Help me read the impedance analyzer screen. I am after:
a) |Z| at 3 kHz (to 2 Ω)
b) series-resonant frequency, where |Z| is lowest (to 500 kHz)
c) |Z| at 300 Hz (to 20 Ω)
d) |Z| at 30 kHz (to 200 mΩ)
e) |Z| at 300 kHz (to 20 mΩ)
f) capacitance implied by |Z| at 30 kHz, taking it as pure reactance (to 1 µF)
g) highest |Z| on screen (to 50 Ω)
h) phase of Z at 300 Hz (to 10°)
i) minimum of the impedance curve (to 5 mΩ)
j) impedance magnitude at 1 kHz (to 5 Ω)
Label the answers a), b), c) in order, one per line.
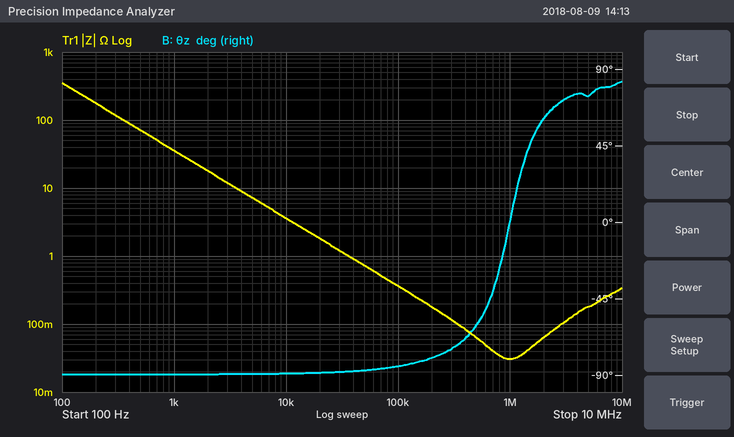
a) 12 Ω
b) 1.0 MHz
c) 120 Ω
d) 1.2 Ω
e) 120 mΩ
f) 4 µF
g) 350 Ω
h) -90°
i) 30 mΩ
j) 35 Ω
